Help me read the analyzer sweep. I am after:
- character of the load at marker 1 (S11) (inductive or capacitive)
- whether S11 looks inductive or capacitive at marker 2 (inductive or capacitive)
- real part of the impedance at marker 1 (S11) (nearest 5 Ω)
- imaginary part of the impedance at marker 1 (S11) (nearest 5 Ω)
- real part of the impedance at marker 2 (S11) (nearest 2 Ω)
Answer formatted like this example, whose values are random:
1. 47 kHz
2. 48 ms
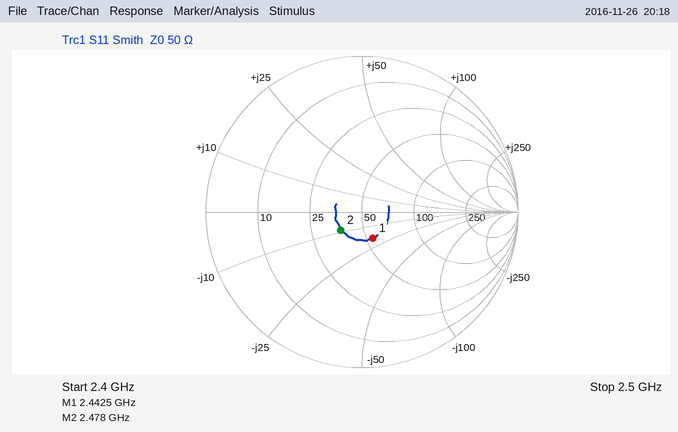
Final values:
1. capacitive
2. capacitive
3. 55 Ω
4. -20 Ω
5. 38 Ω
